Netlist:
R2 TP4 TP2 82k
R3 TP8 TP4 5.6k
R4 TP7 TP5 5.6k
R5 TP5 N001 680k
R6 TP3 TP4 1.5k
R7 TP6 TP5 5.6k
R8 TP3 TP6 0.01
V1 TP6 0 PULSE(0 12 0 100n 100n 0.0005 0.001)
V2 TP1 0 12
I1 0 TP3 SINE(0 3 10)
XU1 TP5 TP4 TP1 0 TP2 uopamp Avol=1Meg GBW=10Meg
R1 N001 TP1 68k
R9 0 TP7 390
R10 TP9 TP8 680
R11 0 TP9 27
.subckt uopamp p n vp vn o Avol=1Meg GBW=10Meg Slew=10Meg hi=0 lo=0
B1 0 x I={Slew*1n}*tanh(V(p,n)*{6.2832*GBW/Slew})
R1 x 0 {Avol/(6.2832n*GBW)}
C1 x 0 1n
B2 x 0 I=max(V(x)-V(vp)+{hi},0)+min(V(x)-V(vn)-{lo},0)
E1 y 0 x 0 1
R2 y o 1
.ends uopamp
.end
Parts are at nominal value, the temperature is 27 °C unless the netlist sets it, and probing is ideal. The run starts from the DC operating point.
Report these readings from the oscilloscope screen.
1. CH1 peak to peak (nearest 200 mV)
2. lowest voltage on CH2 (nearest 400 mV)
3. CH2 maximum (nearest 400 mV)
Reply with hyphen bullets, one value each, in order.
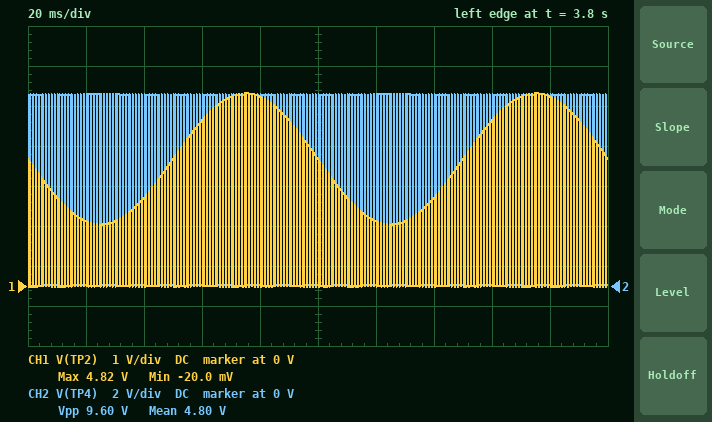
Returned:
- 4.8 V
- 0 V
- 9.6 V
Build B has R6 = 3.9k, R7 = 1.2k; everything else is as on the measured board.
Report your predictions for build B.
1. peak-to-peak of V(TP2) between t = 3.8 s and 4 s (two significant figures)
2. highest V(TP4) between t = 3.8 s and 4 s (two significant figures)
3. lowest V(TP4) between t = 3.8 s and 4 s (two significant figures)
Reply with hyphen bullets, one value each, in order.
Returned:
- 12 V
- 7.6 V
- 16 mV
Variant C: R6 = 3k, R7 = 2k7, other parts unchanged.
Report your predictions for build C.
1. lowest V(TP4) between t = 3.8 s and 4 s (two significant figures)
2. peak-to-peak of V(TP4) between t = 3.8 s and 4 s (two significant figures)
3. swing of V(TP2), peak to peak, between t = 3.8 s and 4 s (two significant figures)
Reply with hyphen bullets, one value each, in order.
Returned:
- 30 mV
- 8.2 V
- 12 V
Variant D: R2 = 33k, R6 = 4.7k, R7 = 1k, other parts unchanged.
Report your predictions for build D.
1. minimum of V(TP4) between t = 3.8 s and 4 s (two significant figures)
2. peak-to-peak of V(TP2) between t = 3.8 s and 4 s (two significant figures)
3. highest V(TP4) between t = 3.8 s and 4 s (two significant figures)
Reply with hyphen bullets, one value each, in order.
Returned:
- 14 mV
- 12 V
- 7.3 V
